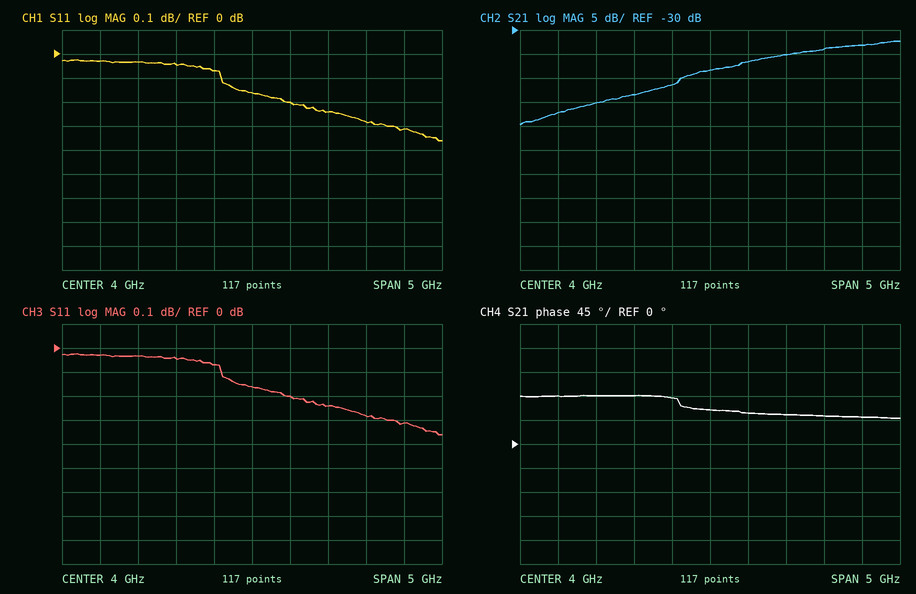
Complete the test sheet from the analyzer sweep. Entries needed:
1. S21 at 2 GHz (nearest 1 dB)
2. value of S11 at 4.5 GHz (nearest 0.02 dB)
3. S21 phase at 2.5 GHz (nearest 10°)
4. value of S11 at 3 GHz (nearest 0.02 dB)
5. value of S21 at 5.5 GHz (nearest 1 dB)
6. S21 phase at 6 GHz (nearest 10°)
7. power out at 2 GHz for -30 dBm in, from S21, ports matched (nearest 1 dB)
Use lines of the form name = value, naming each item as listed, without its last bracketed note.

S21 at 2 GHz = -47 dB
value of S11 at 4.5 GHz = -0.20 dB
S21 phase at 2.5 GHz = 90°
value of S11 at 3 GHz = -0.04 dB
value of S21 at 5.5 GHz = -34 dB
S21 phase at 6 GHz = 50°
power out at 2 GHz for -30 dBm in, from S21, ports matched = -77 dBm
